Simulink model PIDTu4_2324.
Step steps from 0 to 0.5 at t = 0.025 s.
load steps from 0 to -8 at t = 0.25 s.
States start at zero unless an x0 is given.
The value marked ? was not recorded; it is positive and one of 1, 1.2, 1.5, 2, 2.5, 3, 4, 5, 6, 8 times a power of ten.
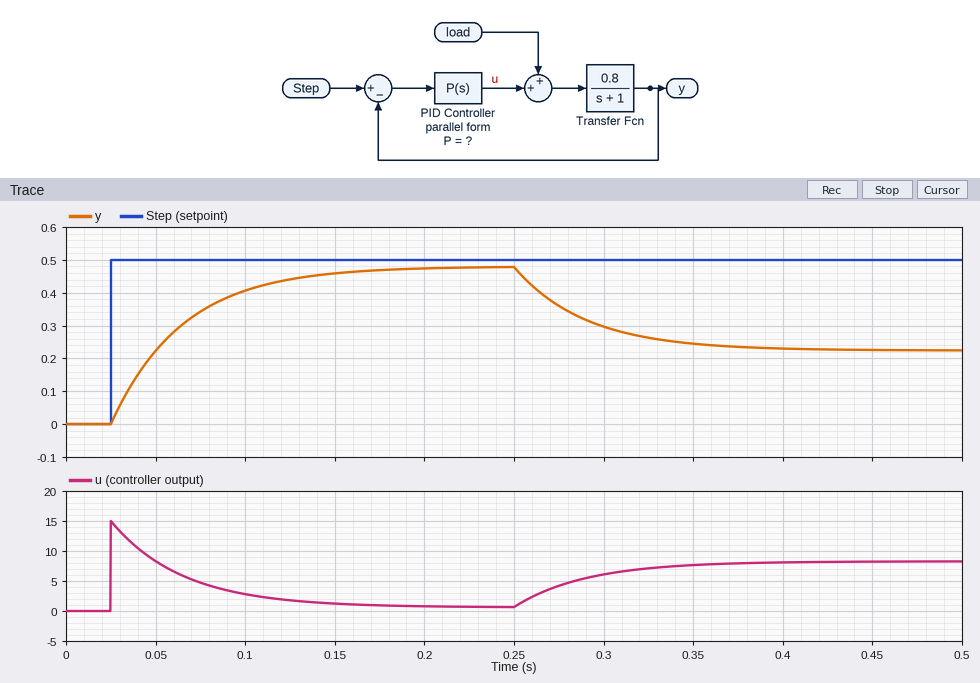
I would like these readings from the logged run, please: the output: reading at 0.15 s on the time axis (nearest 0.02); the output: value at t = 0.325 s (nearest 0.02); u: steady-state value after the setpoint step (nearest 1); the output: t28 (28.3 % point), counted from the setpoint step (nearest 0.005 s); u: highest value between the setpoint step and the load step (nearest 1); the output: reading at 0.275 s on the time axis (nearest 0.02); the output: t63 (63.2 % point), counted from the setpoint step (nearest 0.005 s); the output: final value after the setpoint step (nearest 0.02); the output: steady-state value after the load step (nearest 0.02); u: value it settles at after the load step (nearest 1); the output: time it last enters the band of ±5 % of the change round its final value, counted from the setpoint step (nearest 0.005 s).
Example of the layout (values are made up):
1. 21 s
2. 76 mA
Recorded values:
1. 0.46
2. 0.26
3. 1
4. 0.015 s
5. 15
6. 0.36
7. 0.040 s
8. 0.48
9. 0.22
10. 8
11. 0.120 s
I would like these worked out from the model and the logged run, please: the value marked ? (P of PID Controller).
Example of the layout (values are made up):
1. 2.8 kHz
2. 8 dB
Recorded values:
1. 30
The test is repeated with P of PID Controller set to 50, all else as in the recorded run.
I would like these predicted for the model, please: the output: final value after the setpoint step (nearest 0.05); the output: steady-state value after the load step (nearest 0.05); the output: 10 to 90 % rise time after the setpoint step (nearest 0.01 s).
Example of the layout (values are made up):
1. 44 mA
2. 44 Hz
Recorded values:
1. 0.50
2. 0.35
3. 0.05 s
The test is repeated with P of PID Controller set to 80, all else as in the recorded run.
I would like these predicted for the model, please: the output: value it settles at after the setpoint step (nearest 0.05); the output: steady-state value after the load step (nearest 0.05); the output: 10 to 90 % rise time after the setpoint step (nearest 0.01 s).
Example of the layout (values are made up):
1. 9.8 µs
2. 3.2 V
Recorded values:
1. 0.50
2. 0.40
3. 0.03 s
